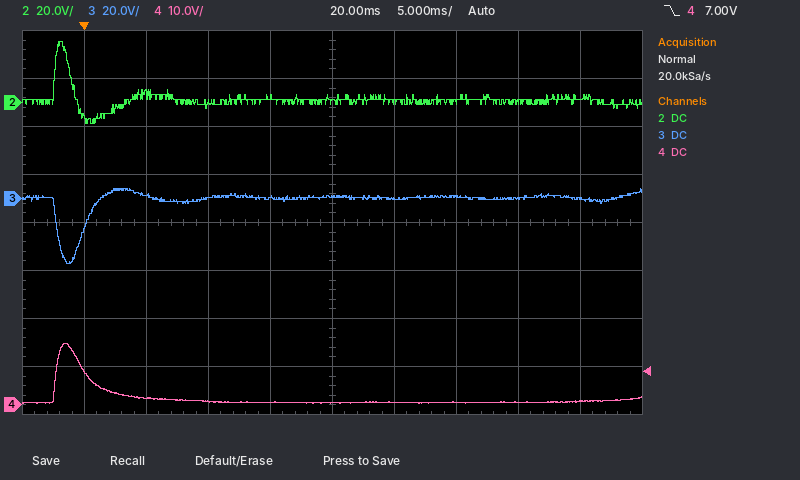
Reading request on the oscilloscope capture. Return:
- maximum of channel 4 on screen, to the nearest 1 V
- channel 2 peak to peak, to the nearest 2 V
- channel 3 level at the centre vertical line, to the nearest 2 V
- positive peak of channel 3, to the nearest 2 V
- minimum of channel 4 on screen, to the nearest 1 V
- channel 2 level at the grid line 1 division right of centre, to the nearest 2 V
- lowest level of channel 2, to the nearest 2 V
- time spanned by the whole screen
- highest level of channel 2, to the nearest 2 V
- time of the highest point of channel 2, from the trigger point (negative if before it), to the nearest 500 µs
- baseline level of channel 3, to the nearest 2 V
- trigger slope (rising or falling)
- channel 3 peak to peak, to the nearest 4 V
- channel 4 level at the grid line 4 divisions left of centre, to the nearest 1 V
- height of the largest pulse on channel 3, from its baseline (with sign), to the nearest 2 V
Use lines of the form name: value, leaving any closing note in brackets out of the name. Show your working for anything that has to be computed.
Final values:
maximum of channel 4 on screen, to the nearest 1 V: 13 V
channel 2 peak to peak, to the nearest 2 V: 26 V − (-8 V) = 34 V
channel 3 level at the centre vertical line, to the nearest 2 V: 0 V
positive peak of channel 3, to the nearest 2 V: 4 V
minimum of channel 4 on screen, to the nearest 1 V: 0 V
channel 2 level at the grid line 1 division right of centre, to the nearest 2 V: 0 V
lowest level of channel 2, to the nearest 2 V: -8 V
time spanned by the whole screen: 50 ms
highest level of channel 2, to the nearest 2 V: 26 V
time of the highest point of channel 2, from the trigger point (negative if before it), to the nearest 500 µs: -2.0 ms
baseline level of channel 3, to the nearest 2 V: 0 V
trigger slope: falling
channel 3 peak to peak, to the nearest 4 V: 32 V
channel 4 level at the grid line 4 divisions left of centre, to the nearest 1 V: 7 V
height of the largest pulse on channel 3, from its baseline (with sign), to the nearest 2 V: -28 V
